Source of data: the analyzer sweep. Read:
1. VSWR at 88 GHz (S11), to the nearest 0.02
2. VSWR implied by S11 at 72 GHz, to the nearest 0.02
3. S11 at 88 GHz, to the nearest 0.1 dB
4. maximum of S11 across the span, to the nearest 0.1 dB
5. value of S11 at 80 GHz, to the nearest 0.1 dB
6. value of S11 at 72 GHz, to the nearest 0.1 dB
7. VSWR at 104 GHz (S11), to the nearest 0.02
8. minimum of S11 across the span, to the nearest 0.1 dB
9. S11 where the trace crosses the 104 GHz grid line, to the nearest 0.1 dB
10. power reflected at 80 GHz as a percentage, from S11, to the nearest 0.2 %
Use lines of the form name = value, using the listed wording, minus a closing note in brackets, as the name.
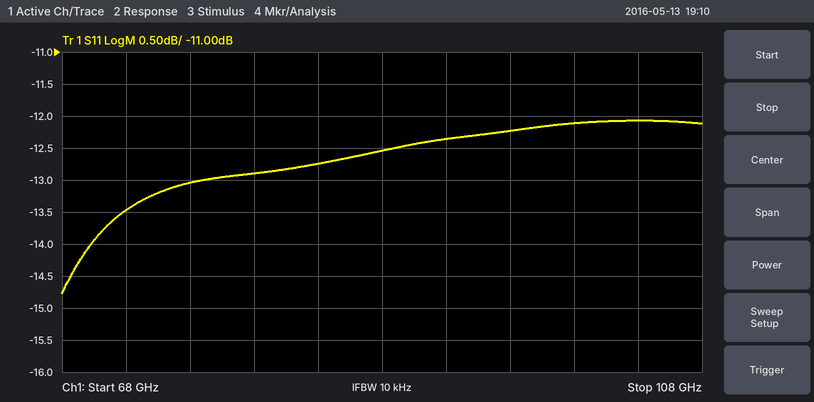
VSWR at 88 GHz (S11), to the nearest 0.02 = 1.62
VSWR implied by S11 at 72 GHz, to the nearest 0.02 = 1.54
S11 at 88 GHz, to the nearest 0.1 dB = -12.5 dB
maximum of S11 across the span, to the nearest 0.1 dB = -12.1 dB
value of S11 at 80 GHz, to the nearest 0.1 dB = -12.9 dB
value of S11 at 72 GHz, to the nearest 0.1 dB = -13.5 dB
VSWR at 104 GHz (S11), to the nearest 0.02 = 1.66
minimum of S11 across the span, to the nearest 0.1 dB = -14.8 dB
S11 where the trace crosses the 104 GHz grid line, to the nearest 0.1 dB = -12.1 dB
power reflected at 80 GHz as a percentage, from S11, to the nearest 0.2 % = 5.2 %
